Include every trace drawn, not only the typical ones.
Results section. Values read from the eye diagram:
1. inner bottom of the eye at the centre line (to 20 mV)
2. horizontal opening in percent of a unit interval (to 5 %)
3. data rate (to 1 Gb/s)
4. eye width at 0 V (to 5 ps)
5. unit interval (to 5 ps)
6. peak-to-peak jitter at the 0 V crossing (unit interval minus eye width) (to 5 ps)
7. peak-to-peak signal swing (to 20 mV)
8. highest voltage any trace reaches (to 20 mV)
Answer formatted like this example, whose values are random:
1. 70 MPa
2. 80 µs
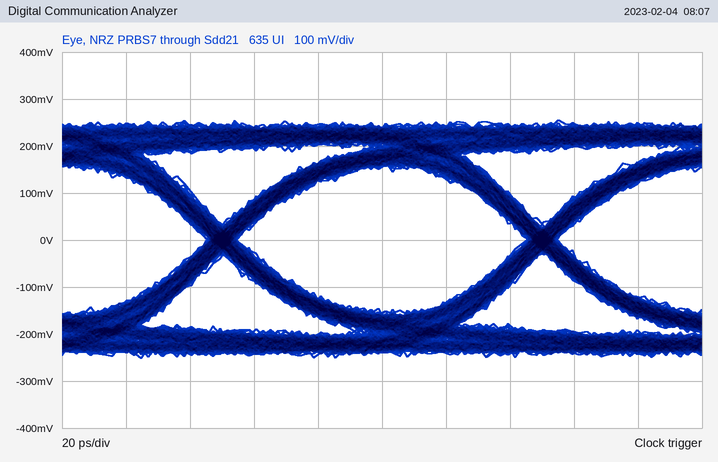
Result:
1. -160 mV
2. 90 %
3. 10 Gb/s
4. 90 ps
5. 100 ps
6. 10 ps
7. 500 mV
8. 260 mV
